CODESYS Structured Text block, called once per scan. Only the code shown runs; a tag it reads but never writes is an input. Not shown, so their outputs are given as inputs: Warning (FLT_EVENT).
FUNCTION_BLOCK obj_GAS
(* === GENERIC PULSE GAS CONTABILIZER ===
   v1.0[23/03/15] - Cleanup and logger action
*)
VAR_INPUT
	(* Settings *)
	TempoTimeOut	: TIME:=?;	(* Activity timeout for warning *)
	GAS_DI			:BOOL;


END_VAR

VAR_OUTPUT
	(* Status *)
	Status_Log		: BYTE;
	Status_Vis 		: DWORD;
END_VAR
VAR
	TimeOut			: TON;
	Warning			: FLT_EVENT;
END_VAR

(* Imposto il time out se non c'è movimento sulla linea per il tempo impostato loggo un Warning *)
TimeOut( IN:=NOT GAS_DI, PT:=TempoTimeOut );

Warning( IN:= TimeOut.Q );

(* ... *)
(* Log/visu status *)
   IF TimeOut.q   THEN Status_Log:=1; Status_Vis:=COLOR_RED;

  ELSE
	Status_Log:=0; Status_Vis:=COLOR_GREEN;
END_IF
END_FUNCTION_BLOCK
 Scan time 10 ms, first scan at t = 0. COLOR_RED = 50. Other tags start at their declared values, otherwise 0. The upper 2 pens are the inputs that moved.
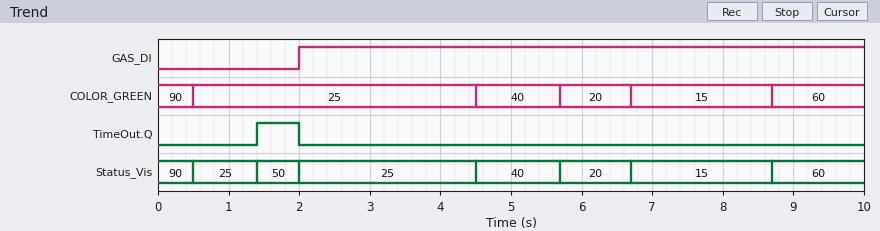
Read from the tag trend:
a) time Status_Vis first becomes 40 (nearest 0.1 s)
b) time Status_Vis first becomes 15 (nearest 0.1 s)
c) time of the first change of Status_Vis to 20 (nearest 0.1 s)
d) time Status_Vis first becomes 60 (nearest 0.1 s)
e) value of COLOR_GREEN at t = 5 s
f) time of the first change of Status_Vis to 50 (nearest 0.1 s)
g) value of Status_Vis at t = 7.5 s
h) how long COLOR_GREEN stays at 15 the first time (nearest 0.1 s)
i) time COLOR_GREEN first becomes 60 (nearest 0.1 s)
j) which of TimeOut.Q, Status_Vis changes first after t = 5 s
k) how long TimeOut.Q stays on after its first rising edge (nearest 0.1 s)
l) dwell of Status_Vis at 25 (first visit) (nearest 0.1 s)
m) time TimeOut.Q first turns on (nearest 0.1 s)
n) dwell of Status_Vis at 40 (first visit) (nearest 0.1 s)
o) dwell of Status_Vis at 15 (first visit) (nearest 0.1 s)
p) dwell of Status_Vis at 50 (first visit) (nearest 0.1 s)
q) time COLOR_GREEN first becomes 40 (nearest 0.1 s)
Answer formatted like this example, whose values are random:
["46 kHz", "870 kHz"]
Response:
["4.5 s", "6.7 s", "5.7 s", "8.7 s", "40", "1.4 s", "15", "2.0 s", "8.7 s", "Status_Vis", "0.6 s", "0.9 s", "1.4 s", "1.2 s", "2.0 s", "0.6 s", "4.5 s"]
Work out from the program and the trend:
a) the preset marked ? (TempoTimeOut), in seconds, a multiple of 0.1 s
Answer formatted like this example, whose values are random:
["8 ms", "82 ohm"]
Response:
["1.4 s"]
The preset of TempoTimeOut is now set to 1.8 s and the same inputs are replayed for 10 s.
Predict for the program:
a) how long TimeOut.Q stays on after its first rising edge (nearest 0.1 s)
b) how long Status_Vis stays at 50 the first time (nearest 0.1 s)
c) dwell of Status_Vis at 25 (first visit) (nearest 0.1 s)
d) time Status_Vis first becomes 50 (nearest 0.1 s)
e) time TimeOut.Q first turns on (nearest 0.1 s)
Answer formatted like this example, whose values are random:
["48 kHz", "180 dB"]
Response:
["0.2 s", "0.2 s", "1.3 s", "1.8 s", "1.8 s"]
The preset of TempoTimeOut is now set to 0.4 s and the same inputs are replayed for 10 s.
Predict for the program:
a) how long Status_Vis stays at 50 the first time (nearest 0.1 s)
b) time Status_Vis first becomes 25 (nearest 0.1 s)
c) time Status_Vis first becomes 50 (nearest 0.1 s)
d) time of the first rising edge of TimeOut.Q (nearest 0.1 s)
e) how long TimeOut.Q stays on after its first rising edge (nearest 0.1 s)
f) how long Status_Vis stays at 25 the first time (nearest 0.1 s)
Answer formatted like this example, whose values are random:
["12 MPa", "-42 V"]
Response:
["1.6 s", "2.0 s", "0.4 s", "0.4 s", "1.6 s", "2.5 s"]
